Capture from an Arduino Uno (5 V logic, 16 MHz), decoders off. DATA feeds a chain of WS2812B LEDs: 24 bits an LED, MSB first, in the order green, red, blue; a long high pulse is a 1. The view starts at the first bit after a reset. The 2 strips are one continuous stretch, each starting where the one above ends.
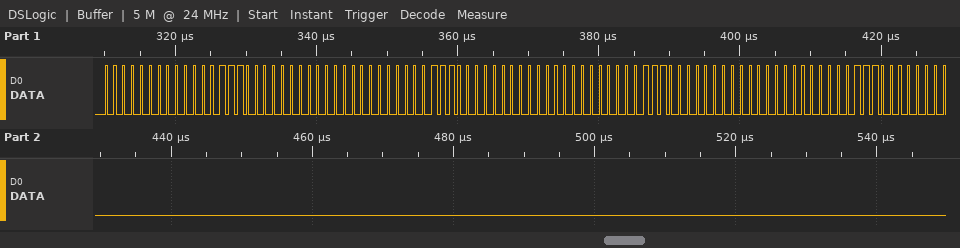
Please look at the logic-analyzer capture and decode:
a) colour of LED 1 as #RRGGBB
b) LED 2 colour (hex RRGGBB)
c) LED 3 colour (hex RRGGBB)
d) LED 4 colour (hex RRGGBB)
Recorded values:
#070000
#070000
#070000
#070000
